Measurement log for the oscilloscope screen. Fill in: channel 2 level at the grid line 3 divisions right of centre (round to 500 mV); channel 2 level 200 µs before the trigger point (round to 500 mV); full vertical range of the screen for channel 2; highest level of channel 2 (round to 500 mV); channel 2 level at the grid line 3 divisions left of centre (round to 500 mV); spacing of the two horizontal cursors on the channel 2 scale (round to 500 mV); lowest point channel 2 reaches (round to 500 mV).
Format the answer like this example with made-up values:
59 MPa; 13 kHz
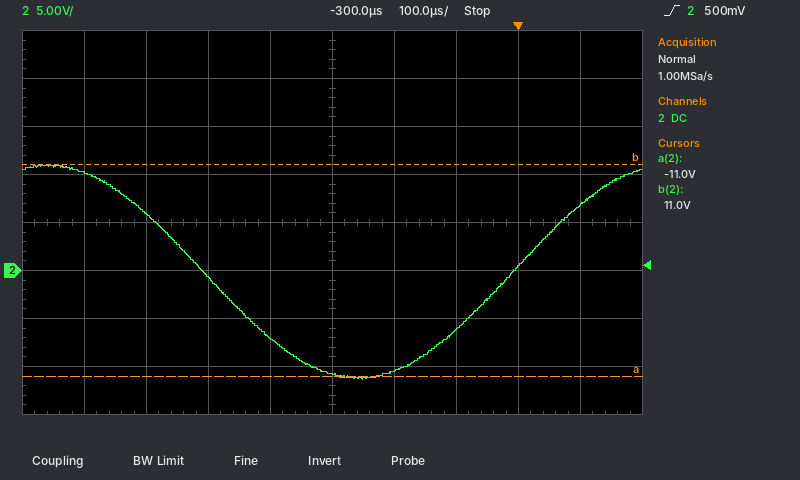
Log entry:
500 mV; -10.5 V; 40 V; 11.0 V; 6.0 V; 22.0 V; -11.5 V
